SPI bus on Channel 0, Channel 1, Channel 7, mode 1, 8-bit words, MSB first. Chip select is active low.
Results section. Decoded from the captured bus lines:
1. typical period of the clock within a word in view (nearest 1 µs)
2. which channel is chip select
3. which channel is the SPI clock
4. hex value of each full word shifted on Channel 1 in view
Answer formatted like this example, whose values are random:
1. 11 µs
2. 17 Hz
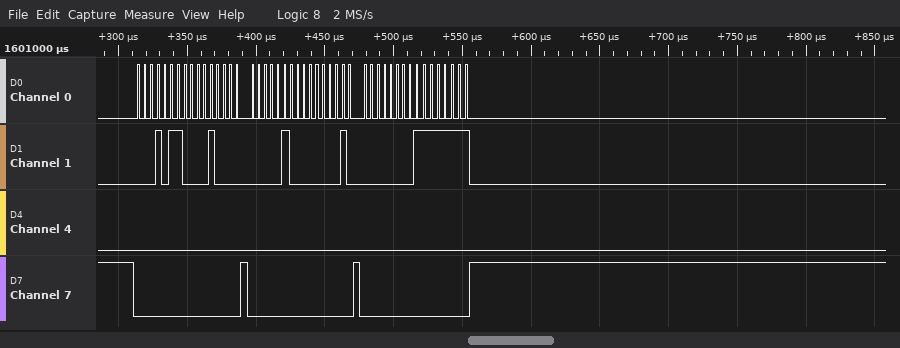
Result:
1. 5 µs
2. Channel 7
3. Channel 0
4. 16, 10, 04, 02, 00, FF
